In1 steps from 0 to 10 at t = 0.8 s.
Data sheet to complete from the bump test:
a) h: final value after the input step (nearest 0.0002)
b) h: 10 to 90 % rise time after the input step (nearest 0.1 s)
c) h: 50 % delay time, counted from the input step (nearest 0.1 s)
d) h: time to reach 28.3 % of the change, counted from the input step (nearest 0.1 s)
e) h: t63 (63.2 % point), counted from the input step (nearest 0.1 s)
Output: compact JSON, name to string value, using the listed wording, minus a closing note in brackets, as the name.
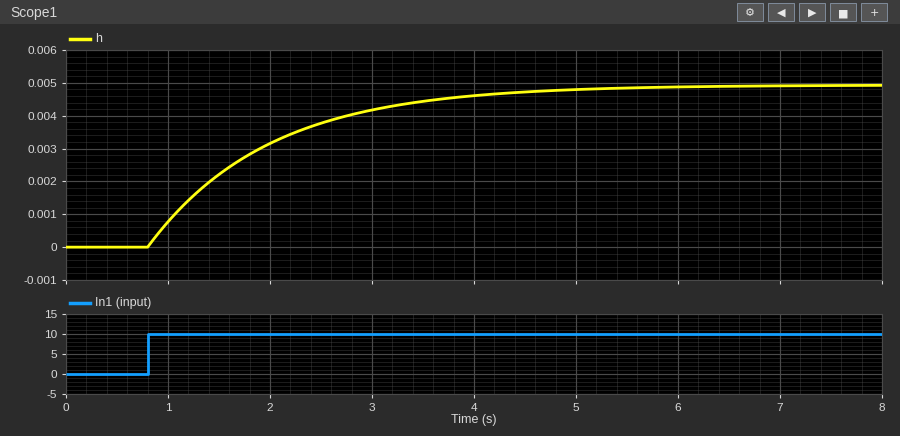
{"h: final value after the input step": "0.0050", "h: 10 to 90 % rise time after the input step": "2.6 s", "h: 50 % delay time, counted from the input step": "0.8 s", "h: time to reach 28.3 % of the change, counted from the input step": "0.4 s", "h: t63 (63.2 % point), counted from the input step": "1.2 s"}
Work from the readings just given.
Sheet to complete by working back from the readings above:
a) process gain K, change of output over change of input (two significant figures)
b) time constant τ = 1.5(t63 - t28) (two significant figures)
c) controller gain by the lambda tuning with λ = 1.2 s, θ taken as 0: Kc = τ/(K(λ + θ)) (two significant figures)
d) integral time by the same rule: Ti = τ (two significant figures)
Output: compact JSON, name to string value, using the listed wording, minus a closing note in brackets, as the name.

{"process gain K, change of output over change of input": "0.00050", "time constant τ = 1.5(t63 - t28)": "1.2 s", "controller gain by the lambda tuning with λ = 1.2 s, θ taken as 0: Kc = τ/(K(λ + θ))": "2000", "integral time by the same rule: Ti = τ": "1.2 s"}
